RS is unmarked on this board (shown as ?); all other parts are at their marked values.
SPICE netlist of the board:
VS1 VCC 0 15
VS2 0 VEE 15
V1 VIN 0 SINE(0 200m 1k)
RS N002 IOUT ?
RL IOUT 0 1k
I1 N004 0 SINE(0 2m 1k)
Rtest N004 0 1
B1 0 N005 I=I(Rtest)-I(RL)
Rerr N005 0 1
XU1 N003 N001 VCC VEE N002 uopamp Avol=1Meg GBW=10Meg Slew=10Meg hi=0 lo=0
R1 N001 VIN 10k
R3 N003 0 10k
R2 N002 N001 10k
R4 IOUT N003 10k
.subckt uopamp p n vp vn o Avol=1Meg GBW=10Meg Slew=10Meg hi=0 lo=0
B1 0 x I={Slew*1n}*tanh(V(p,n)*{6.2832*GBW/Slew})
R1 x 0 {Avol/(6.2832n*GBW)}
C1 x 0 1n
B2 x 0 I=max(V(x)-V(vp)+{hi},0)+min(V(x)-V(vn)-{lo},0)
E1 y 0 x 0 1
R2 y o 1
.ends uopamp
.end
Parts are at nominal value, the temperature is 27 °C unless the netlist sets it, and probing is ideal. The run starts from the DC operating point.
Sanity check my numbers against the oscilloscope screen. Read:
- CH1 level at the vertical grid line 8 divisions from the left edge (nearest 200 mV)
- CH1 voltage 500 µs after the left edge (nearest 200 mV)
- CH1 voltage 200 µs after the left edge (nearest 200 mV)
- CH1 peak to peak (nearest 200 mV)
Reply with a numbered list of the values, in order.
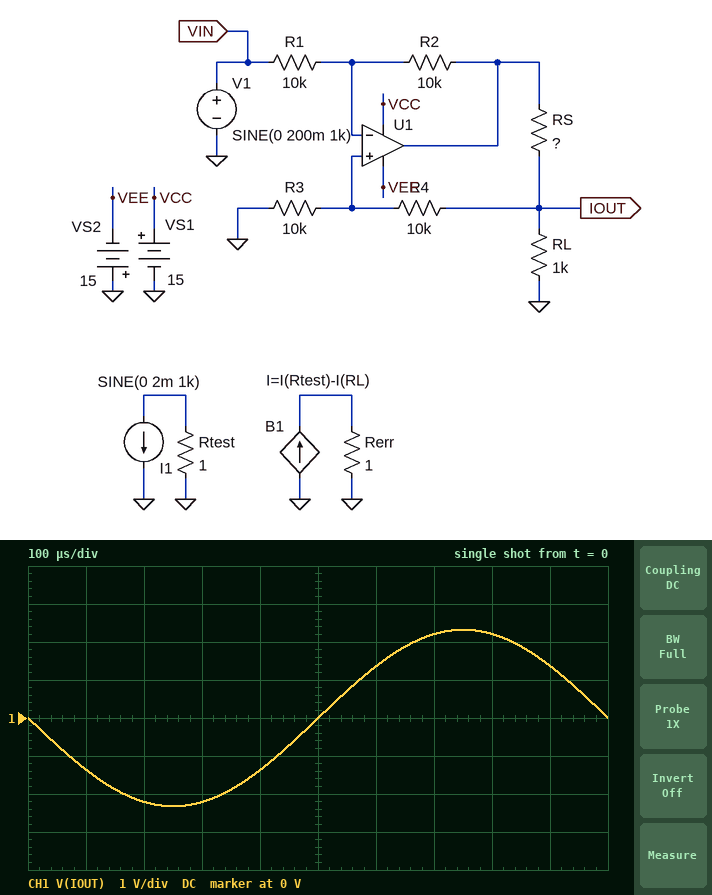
1. 2.2 V
2. 0 V
3. -2.2 V
4. 4.6 V
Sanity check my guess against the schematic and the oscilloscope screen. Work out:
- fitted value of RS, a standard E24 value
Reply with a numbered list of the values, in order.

1. 82 Ω
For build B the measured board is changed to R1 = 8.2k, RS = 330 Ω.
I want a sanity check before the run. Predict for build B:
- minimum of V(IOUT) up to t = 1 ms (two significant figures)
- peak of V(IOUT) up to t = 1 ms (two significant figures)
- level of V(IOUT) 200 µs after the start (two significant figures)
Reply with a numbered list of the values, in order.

1. -1.0 V
2. 1.0 V
3. -980 mV
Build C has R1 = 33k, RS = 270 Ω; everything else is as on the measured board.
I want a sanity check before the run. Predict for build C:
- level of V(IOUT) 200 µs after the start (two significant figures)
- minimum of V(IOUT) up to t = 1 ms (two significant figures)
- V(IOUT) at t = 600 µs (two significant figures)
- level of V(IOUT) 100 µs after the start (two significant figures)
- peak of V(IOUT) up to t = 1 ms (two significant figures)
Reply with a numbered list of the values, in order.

1. -91 mV
2. -96 mV
3. 56 mV
4. -56 mV
5. 96 mV
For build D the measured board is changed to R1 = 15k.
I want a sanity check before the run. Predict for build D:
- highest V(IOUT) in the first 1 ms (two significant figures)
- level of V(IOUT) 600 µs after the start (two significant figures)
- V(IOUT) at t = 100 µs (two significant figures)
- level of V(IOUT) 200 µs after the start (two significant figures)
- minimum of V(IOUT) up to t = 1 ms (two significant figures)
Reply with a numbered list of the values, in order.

1. 530 mV
2. 310 mV
3. -310 mV
4. -500 mV
5. -530 mV
